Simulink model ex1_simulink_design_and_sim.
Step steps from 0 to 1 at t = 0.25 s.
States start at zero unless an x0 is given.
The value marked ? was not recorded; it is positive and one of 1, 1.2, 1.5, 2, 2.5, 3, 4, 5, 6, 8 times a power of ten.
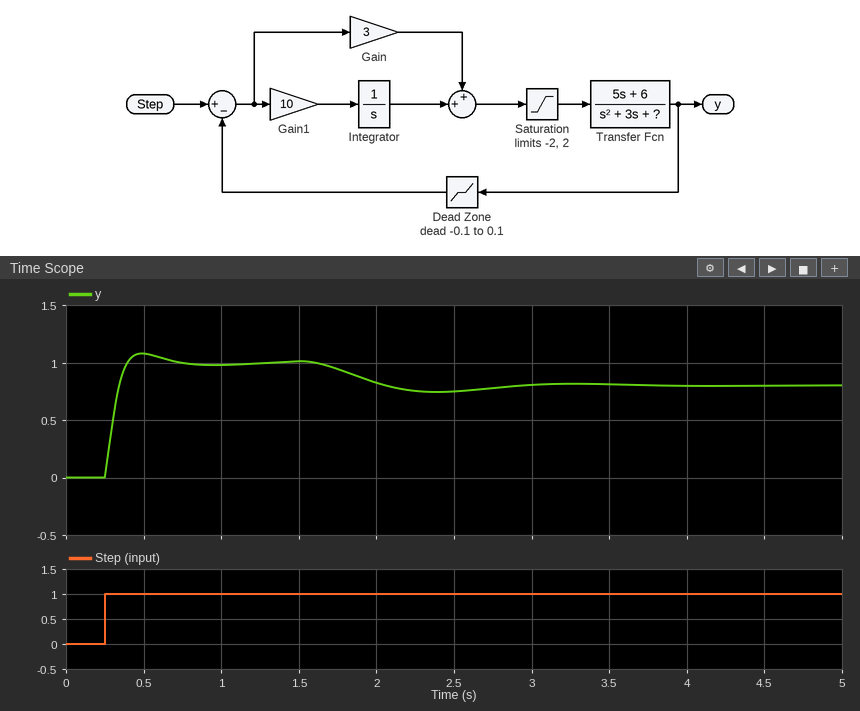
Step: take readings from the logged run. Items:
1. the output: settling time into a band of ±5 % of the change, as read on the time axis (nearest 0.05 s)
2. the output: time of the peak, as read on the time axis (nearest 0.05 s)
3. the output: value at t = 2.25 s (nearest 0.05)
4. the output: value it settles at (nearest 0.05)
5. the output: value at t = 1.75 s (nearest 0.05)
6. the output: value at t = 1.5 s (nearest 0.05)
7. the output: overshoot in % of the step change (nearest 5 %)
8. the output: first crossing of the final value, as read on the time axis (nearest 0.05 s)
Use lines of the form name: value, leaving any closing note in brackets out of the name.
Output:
the output: settling time into a band of ±5 % of the change, as read on the time axis: 2.60 s
the output: time of the peak, as read on the time axis: 0.50 s
the output: value at t = 2.25 s: 0.75
the output: value it settles at: 0.80
the output: value at t = 1.75 s: 0.95
the output: value at t = 1.5 s: 1.00
the output: overshoot in % of the step change: 35 %
the output: first crossing of the final value, as read on the time axis: 0.35 s
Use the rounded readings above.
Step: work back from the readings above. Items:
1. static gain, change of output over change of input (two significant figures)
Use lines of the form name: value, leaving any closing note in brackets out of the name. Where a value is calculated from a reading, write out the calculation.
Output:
static gain, change of output over change of input: (0.8 - 0) / (1 - 0) = 0.80
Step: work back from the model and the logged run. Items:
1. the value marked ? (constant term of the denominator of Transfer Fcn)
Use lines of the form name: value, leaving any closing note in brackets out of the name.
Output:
the value marked ?: 15
